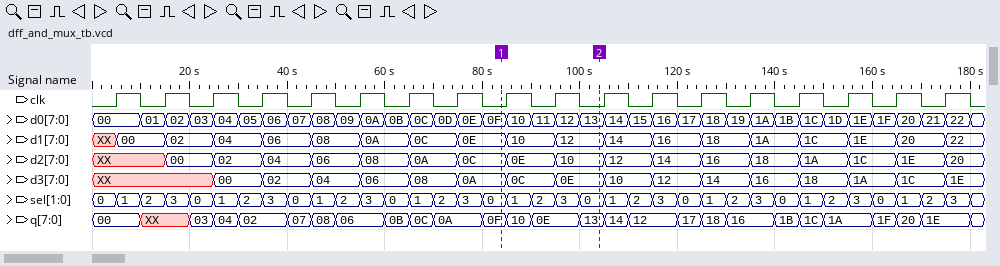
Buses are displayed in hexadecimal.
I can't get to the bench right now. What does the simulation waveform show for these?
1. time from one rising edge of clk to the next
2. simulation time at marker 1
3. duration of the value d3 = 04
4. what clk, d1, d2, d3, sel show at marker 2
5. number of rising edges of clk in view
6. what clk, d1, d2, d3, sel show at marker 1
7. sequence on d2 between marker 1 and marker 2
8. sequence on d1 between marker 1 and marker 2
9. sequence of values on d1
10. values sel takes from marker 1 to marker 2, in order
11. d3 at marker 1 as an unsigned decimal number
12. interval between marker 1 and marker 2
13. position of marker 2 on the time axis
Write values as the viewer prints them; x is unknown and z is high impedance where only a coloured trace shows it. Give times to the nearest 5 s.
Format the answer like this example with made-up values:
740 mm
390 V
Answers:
10 s
85 s
10 s
clk=0, d1=12, d2=10, d3=0E, sel=0
18
clk=0, d1=0E, d2=0C, d3=0A, sel=0
0C, 0E, 10
0E, 10, 12
XX, 00, 02, 04, 06, 08, 0A, 0C, 0E, 10, 12, 14, 16, 18, 1A, 1C, 1E, 20, 22
0, 1, 2, 3, 0
10
20 s
105 s
